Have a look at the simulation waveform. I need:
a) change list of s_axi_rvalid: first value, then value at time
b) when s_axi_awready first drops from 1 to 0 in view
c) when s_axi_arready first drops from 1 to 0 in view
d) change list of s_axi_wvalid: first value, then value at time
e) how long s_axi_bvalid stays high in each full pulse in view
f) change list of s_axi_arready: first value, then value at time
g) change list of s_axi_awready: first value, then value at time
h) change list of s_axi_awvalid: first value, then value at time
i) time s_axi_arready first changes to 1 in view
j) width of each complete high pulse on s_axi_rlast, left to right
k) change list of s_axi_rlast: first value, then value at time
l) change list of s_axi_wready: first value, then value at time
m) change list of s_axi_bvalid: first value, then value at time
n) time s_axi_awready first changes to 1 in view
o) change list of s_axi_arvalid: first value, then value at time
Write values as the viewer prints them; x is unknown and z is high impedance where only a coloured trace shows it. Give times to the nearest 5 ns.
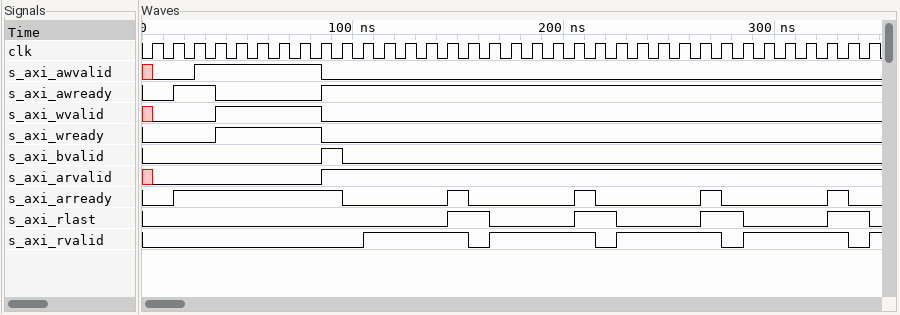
0, 1 at 105 ns, 0 at 155 ns, 1 at 165 ns, 0 at 215 ns, 1 at 225 ns, 0 at 275 ns, 1 at 285 ns, 0 at 335 ns, 1 at 345 ns
35 ns
95 ns
x, 0 at 5 ns, 1 at 35 ns, 0 at 85 ns
10 ns
0, 1 at 15 ns, 0 at 95 ns, 1 at 145 ns, 0 at 155 ns, 1 at 205 ns, 0 at 215 ns, 1 at 265 ns, 0 at 275 ns, 1 at 325 ns, 0 at 335 ns
0, 1 at 15 ns, 0 at 35 ns, 1 at 85 ns
x, 0 at 5 ns, 1 at 25 ns, 0 at 85 ns
15 ns
20 ns, 20 ns, 20 ns, 20 ns
0, 1 at 145 ns, 0 at 165 ns, 1 at 205 ns, 0 at 225 ns, 1 at 265 ns, 0 at 285 ns, 1 at 325 ns, 0 at 345 ns
0, 1 at 35 ns, 0 at 85 ns
0, 1 at 85 ns, 0 at 95 ns
15 ns
x, 0 at 5 ns, 1 at 85 ns
